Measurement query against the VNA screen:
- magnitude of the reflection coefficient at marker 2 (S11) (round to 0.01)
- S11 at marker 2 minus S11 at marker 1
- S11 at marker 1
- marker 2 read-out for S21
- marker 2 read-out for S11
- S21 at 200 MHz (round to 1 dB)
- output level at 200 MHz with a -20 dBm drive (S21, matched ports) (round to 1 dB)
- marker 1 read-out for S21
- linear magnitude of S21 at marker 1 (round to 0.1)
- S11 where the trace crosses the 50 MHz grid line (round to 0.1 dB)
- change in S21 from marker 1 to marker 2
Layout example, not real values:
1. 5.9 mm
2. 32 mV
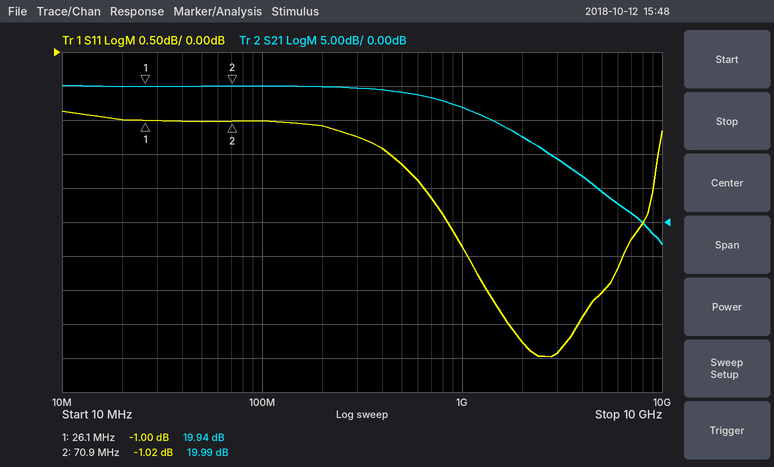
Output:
1. 0.89
2. -0.02 dB
3. -1.00 dB
4. 19.99 dB
5. -1.02 dB
6. 20 dB
7. 0 dBm
8. 19.94 dB
9. 9.9
10. -1.0 dB
11. 0.05 dB
